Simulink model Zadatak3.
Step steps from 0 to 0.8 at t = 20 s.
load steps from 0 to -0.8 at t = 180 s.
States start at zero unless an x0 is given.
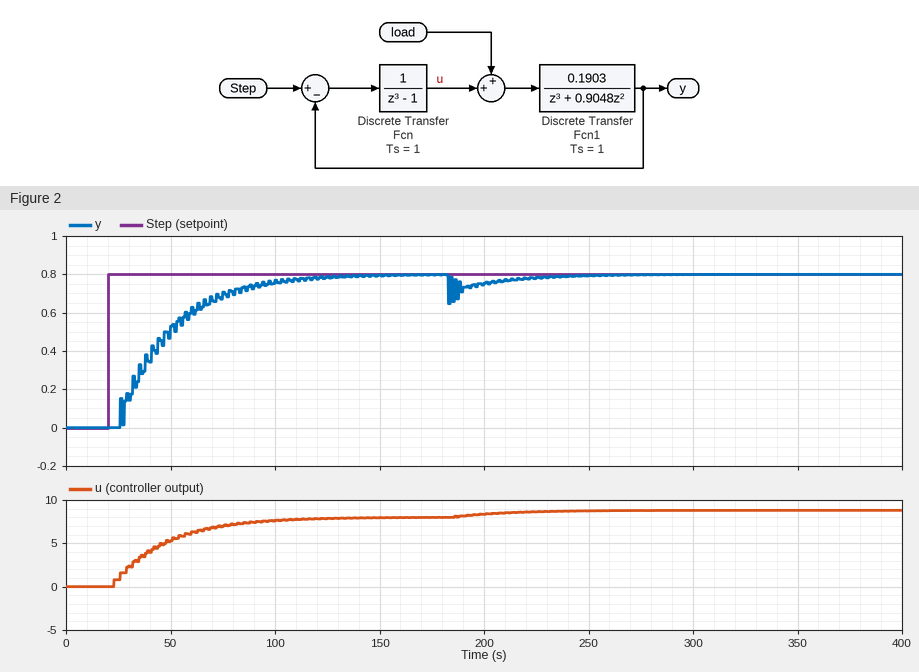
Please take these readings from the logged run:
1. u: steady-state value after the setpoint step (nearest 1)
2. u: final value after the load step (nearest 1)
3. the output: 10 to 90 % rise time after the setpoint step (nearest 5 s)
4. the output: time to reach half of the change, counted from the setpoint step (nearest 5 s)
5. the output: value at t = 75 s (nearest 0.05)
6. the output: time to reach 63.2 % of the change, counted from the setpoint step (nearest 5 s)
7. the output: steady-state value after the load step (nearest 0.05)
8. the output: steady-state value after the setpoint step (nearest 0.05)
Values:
8
9
55 s
20 s
0.70
30 s
0.80
0.80
